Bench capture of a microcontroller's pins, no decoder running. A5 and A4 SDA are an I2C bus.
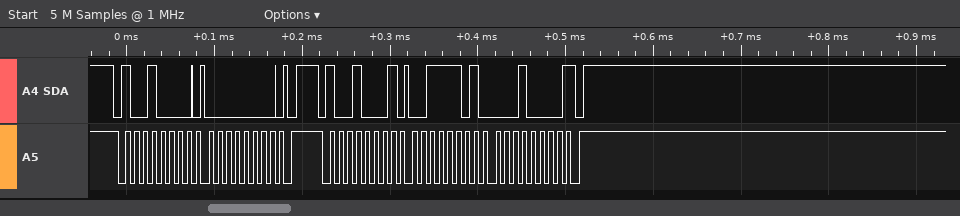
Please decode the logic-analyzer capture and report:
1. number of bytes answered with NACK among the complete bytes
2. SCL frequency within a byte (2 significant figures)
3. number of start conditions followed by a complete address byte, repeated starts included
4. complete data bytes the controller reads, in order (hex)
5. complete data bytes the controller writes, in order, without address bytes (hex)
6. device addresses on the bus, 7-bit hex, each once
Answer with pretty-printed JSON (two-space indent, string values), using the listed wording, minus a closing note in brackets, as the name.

{
  "number of bytes answered with NACK among the complete bytes": "1",
  "SCL frequency within a byte": "100 kHz",
  "number of start conditions followed by a complete address byte, repeated starts included": "2",
  "complete data bytes the controller reads, in order": "3D 10",
  "complete data bytes the controller writes, in order, without address bytes": "00",
  "device addresses on the bus, 7-bit hex, each once": "0x48"
}
